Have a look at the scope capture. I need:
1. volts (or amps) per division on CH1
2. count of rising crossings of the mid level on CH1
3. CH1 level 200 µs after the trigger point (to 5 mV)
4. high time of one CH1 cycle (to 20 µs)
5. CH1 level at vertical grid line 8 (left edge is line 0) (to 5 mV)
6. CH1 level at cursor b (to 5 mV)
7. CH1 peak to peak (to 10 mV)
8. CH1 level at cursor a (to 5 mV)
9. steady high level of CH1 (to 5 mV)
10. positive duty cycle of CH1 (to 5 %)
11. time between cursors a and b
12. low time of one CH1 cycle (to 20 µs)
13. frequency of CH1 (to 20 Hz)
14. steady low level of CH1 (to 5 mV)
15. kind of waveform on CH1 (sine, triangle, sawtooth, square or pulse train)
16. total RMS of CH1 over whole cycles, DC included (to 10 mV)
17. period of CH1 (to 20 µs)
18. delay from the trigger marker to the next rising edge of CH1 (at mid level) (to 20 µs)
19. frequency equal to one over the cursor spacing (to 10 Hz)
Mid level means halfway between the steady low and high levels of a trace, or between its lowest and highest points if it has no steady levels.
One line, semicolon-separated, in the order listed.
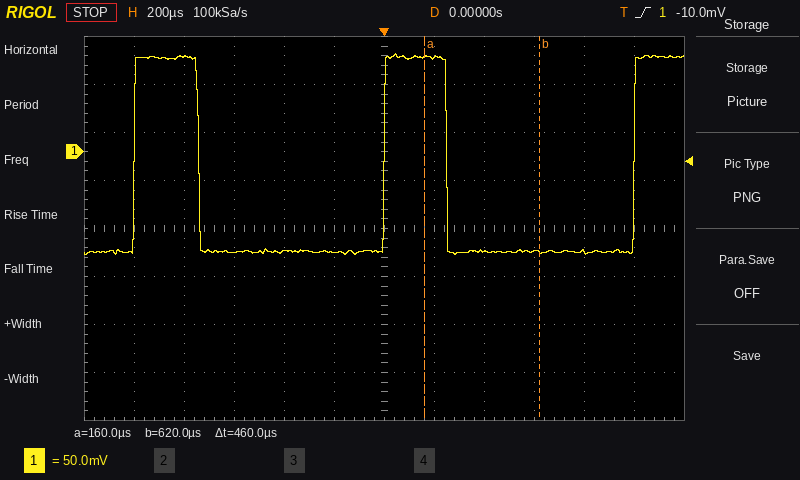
50 mV; 3; 100 mV; 260 µs; -105 mV; -105 mV; 210 mV; 100 mV; 100 mV; 25 %; 460 µs; 740 µs; 1.00 kHz; -105 mV; pulse train; 100 mV; 1.00 ms; 1.00 ms; 2.17 kHz
